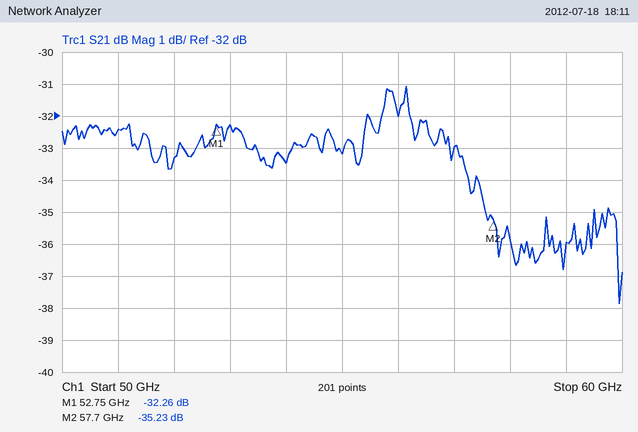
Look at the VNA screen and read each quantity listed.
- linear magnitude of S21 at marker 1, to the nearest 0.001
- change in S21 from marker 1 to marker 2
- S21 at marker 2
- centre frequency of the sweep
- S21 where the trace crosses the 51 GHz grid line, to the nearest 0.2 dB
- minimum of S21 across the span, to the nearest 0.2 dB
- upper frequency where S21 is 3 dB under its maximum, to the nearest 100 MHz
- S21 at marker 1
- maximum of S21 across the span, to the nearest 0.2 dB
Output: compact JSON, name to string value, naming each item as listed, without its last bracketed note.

{"linear magnitude of S21 at marker 1, to the nearest 0.001": "0.024", "change in S21 from marker 1 to marker 2": "-2.97 dB", "S21 at marker 2": "-35.23 dB", "centre frequency of the sweep": "55 GHz", "S21 where the trace crosses the 51 GHz grid line, to the nearest 0.2 dB": "-32.4 dB", "minimum of S21 across the span, to the nearest 0.2 dB": "-37.8 dB", "upper frequency where S21 is 3 dB under its maximum, to the nearest 100 MHz": "57.3 GHz", "S21 at marker 1": "-32.26 dB", "maximum of S21 across the span, to the nearest 0.2 dB": "-31.0 dB"}
